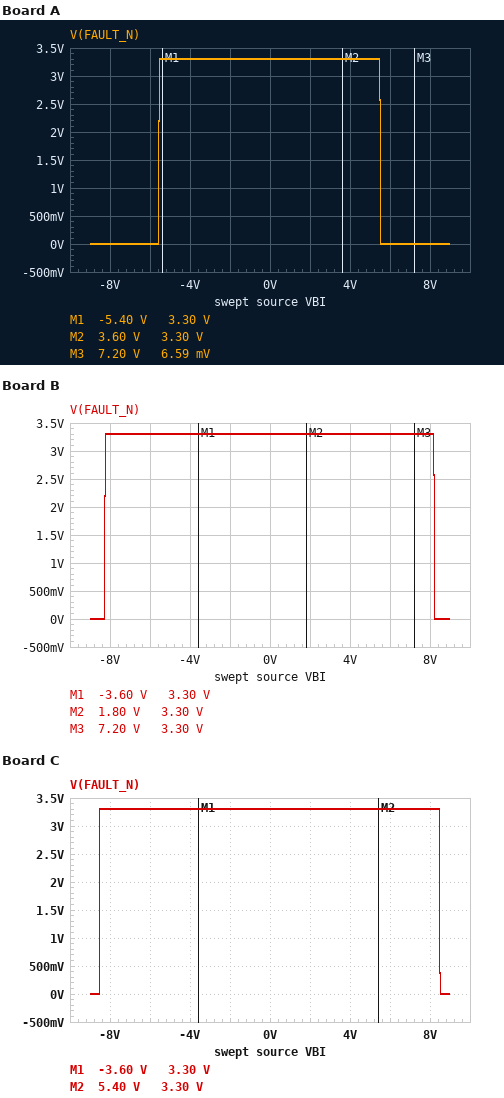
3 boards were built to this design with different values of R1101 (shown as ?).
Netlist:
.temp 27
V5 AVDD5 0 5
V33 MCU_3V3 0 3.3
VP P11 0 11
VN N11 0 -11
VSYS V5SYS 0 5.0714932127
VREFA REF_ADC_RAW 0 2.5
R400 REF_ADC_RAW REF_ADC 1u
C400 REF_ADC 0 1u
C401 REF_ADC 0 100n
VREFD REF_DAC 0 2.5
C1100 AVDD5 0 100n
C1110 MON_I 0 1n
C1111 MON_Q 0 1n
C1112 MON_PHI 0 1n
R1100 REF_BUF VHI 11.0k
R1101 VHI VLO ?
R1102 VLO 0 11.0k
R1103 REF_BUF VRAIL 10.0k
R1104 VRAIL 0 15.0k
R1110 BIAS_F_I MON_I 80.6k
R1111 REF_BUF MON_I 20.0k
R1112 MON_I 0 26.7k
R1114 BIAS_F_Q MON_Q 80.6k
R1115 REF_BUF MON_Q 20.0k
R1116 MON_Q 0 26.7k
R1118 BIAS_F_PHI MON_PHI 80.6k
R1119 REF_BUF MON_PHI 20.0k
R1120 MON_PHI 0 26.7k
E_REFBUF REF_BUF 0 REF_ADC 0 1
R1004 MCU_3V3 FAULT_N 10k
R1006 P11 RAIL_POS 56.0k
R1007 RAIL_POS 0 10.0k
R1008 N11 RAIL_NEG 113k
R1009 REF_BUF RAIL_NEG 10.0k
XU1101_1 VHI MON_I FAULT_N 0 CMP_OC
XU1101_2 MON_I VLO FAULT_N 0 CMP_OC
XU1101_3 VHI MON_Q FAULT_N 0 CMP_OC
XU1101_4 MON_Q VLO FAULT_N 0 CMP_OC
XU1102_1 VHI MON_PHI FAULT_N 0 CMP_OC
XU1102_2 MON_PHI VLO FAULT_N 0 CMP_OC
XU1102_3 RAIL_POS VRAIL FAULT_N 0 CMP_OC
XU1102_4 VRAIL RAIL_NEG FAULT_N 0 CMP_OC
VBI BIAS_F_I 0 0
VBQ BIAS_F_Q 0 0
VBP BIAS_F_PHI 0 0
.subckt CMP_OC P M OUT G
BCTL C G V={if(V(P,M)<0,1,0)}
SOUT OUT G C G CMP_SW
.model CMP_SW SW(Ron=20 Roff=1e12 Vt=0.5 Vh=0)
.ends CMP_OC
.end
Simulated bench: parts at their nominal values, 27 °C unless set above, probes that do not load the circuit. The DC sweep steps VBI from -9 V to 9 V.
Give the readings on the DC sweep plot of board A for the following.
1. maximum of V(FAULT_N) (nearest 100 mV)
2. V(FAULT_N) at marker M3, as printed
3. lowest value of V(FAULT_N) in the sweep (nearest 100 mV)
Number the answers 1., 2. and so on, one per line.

1. 3.3 V
2. 6.59 mV
3. 0 V
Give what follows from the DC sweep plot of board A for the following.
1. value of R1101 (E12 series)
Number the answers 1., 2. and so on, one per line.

1. 27 kΩ
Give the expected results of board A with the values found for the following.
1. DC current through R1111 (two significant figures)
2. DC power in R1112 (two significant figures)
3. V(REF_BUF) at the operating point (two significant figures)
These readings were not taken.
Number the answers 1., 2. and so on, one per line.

1. 62 µA
2. 59 µW
3. 2.5 V
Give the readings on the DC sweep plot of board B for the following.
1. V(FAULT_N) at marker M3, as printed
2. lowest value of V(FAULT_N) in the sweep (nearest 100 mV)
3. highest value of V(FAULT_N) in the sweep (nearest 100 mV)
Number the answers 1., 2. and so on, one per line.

1. 3.30 V
2. 0 V
3. 3.3 V
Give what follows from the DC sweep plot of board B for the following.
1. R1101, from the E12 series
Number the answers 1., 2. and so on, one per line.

1. 100 kΩ
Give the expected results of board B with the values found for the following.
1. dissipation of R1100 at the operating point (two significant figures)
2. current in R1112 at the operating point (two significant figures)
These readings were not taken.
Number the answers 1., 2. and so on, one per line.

1. 4.6 µW
2. 47 µA
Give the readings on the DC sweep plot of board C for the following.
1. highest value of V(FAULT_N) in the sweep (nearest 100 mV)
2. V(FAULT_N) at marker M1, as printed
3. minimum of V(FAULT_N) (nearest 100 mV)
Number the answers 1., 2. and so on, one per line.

1. 3.3 V
2. 3.30 V
3. 0 V
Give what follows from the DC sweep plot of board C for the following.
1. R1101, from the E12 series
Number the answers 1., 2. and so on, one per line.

1. 120 kΩ
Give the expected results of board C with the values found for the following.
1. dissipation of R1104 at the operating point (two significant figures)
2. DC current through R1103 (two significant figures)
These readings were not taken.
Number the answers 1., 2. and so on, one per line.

1. 150 µW
2. 100 µA
